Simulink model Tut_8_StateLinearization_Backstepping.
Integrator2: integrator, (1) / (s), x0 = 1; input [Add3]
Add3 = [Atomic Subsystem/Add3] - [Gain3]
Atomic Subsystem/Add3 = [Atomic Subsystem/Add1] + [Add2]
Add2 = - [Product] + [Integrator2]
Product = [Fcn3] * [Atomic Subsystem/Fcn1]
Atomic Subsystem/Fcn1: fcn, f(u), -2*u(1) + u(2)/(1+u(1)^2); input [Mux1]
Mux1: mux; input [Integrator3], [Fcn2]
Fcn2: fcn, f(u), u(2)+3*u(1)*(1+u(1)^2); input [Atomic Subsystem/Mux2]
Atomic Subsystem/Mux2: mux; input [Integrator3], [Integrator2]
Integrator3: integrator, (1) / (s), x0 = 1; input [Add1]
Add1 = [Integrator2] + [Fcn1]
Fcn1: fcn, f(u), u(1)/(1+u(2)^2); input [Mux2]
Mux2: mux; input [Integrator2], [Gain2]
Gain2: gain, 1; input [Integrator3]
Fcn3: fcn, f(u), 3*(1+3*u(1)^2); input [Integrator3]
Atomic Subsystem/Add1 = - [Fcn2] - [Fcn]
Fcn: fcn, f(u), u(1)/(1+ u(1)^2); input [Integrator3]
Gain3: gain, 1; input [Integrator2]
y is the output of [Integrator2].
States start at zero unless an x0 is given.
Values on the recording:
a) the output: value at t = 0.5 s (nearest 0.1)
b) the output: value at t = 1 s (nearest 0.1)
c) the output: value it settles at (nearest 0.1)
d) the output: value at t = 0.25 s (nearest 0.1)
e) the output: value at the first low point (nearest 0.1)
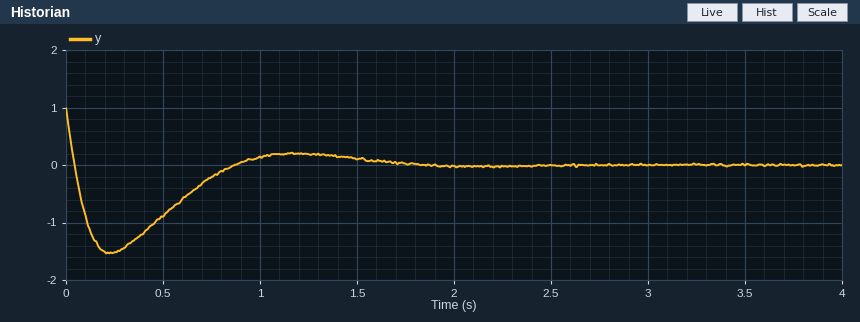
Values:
-0.9
0.1
0.0
-1.5
-1.5
